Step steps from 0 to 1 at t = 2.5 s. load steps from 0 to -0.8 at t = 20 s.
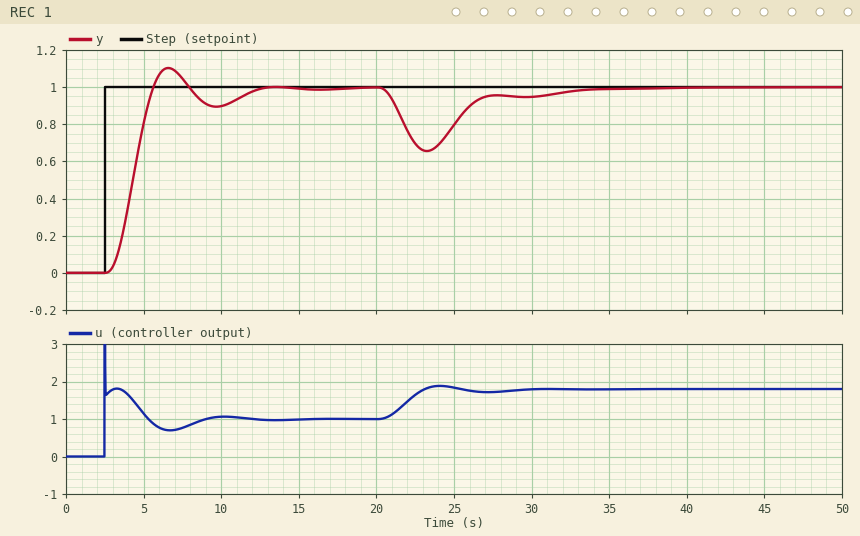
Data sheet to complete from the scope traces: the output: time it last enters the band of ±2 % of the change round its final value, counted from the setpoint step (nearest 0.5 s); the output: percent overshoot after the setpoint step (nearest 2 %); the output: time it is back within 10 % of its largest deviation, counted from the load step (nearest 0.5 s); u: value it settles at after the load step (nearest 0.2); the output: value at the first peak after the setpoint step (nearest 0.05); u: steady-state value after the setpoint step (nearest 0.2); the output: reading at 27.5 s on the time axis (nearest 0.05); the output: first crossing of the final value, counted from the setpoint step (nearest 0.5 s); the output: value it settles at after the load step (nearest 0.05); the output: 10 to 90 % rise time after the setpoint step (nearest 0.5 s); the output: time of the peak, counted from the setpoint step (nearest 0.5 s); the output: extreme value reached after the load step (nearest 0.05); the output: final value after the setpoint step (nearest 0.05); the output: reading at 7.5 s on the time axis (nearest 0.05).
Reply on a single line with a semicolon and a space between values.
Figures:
9.5 s; 10 %; 11.5 s; 1.8; 1.10; 1.0; 0.95; 3.0 s; 1.00; 2.0 s; 4.0 s; 0.65; 1.00; 1.05
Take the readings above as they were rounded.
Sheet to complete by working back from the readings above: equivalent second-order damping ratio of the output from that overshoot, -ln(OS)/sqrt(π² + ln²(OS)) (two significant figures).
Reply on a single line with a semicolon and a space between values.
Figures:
0.59
